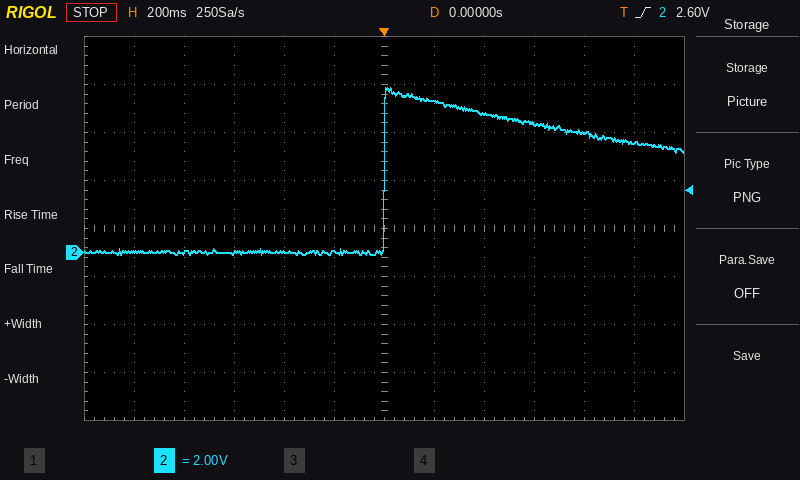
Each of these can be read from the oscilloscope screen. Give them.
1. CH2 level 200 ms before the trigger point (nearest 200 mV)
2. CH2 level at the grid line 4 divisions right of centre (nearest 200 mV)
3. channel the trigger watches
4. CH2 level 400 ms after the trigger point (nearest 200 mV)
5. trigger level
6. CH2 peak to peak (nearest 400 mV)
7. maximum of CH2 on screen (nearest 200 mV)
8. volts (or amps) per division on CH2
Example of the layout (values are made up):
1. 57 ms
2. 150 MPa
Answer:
1. 0.0 V
2. 5.0 V
3. CH2
4. 5.8 V
5. 2.60 V
6. 6.8 V
7. 6.8 V
8. 2 V
